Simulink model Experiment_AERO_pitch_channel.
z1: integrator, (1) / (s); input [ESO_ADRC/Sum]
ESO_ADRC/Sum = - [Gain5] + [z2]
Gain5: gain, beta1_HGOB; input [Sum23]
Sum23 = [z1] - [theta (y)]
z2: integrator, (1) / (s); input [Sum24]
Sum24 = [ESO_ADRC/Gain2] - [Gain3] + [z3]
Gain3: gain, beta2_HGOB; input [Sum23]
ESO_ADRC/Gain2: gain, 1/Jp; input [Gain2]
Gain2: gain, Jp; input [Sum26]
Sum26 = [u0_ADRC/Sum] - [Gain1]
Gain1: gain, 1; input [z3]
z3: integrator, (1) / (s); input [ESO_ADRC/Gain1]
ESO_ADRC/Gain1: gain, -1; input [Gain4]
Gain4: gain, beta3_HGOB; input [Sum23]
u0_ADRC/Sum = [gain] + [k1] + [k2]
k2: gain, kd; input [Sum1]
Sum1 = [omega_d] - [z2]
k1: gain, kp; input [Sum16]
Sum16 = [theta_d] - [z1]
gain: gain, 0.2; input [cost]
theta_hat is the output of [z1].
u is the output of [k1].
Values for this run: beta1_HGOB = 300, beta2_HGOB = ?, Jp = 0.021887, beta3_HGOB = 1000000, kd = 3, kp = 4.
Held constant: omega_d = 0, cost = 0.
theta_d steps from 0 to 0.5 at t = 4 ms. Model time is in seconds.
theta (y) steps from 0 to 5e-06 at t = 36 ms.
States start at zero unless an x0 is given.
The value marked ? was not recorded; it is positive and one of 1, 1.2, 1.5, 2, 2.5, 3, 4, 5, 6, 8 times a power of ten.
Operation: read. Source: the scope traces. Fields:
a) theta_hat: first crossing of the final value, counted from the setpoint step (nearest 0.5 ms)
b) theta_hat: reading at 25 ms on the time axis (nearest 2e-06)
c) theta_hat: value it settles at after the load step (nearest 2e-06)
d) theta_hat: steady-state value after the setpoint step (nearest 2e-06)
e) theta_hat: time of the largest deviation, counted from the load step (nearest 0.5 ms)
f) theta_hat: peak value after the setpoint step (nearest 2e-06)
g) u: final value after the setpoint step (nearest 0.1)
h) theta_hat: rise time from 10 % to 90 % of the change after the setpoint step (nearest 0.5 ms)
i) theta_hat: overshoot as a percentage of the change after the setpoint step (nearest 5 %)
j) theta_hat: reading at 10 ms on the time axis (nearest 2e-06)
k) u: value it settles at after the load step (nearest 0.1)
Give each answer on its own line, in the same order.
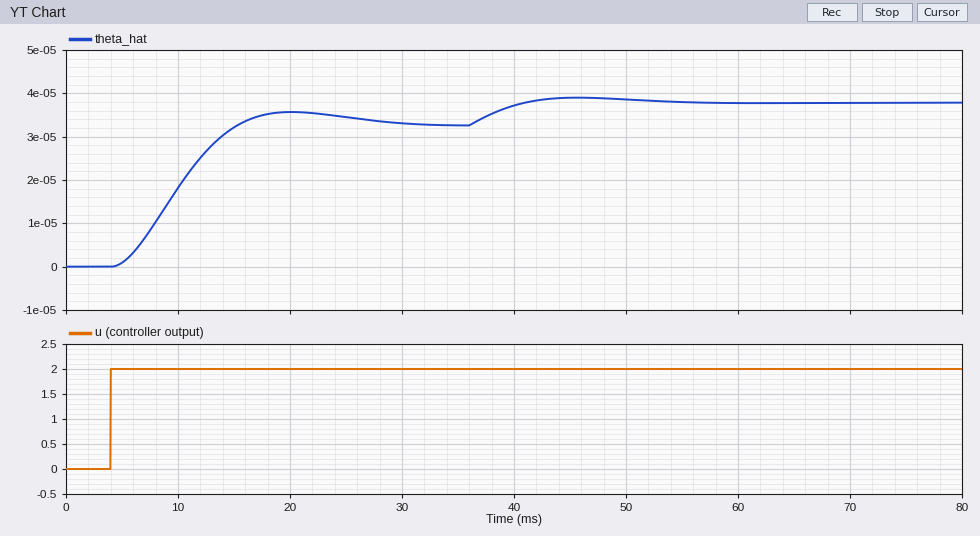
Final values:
11.5 ms
0.000034
0.000038
0.000032
9.5 ms
0.000036
2.0
7.5 ms
10 %
0.000018
2.0
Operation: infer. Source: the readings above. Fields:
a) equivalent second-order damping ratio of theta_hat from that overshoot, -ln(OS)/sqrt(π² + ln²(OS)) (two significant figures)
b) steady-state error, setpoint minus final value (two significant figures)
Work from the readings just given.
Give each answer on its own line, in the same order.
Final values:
0.59
0.50
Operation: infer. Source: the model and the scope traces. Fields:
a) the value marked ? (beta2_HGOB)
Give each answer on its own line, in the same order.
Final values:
60000
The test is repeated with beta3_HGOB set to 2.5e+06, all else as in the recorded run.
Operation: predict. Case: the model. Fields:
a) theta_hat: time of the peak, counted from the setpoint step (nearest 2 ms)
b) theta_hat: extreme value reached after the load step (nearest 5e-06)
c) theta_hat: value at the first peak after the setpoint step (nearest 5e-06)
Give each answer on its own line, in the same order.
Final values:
16 ms
0.000040
0.000035
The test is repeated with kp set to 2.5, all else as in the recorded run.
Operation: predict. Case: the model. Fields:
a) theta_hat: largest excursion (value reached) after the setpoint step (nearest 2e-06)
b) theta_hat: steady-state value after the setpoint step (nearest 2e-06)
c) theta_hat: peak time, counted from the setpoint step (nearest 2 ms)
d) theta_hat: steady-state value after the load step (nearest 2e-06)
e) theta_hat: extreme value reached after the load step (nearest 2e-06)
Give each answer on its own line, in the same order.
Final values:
0.000022
0.000020
16 ms
0.000026
0.000026
